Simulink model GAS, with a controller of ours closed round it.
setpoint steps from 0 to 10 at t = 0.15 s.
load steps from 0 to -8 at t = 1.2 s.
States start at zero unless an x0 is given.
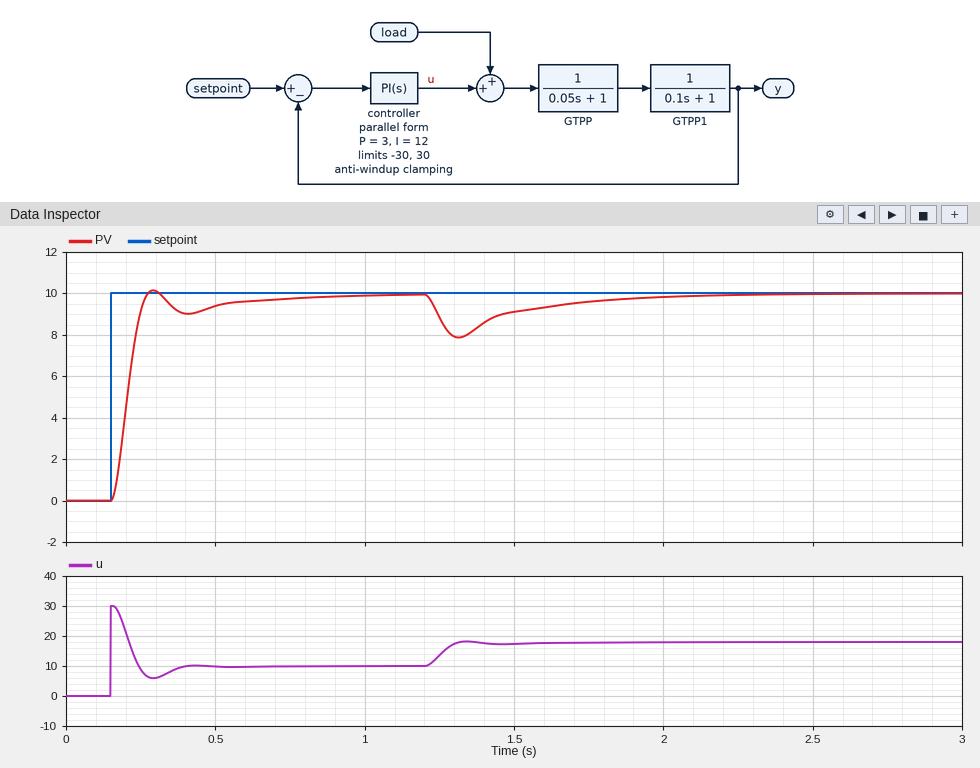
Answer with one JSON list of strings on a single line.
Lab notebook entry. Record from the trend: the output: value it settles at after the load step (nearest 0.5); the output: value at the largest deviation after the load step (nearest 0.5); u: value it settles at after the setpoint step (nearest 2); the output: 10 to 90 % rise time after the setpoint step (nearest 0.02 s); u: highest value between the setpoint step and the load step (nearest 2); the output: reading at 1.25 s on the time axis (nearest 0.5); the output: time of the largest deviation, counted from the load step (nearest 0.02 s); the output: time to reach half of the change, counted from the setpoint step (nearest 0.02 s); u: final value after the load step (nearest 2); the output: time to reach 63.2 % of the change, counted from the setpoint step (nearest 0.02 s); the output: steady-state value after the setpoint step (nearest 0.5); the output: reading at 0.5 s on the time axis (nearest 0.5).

["10.0", "8.0", "10", "0.08 s", "30", "9.0", "0.12 s", "0.06 s", "18", "0.06 s", "10.0", "9.5"]
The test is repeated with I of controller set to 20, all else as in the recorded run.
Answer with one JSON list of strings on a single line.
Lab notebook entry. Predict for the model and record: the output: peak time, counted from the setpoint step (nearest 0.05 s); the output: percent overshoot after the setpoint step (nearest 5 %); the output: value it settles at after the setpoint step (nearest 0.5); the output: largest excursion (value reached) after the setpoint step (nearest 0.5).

["0.15 s", "10 %", "10.0", "11.0"]
